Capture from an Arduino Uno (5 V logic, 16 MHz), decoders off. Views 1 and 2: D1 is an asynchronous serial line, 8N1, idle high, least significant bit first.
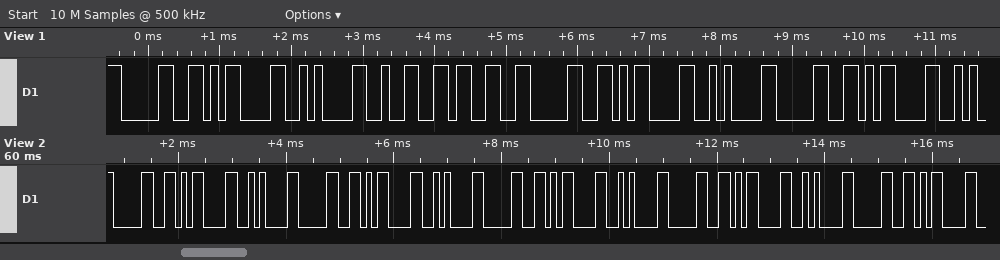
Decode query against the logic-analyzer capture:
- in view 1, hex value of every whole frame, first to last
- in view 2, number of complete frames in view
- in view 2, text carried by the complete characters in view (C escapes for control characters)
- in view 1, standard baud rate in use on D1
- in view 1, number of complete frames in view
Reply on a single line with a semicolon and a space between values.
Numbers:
30 0D 0A 32 33 30 0D 0A 30 0D; 14; "0\r\n0\r\n0\r\n0\r\n0\r"; 9600 baud; 10
